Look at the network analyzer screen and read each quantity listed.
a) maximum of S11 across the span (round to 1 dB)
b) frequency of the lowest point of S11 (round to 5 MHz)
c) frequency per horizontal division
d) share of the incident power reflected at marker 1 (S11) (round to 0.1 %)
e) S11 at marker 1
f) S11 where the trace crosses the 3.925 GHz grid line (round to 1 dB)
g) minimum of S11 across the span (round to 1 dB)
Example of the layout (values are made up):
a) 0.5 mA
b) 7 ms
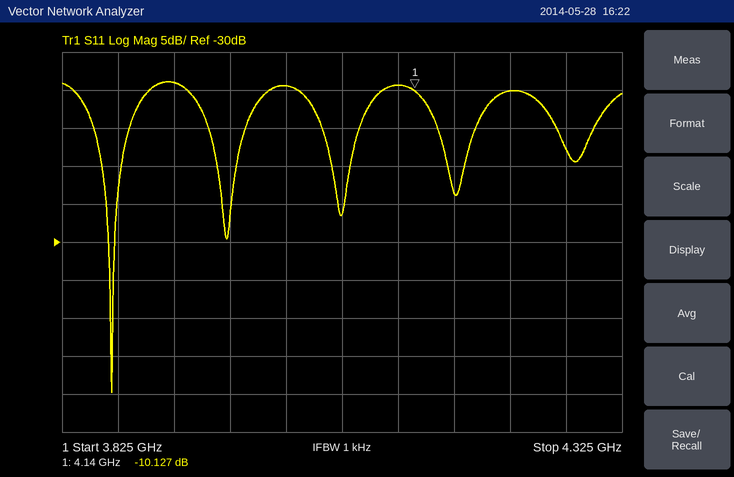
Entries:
a) -9 dB
b) 3.870 GHz
c) 50 MHz
d) 9.7 %
e) -10.127 dB
f) -9 dB
g) -50 dB
